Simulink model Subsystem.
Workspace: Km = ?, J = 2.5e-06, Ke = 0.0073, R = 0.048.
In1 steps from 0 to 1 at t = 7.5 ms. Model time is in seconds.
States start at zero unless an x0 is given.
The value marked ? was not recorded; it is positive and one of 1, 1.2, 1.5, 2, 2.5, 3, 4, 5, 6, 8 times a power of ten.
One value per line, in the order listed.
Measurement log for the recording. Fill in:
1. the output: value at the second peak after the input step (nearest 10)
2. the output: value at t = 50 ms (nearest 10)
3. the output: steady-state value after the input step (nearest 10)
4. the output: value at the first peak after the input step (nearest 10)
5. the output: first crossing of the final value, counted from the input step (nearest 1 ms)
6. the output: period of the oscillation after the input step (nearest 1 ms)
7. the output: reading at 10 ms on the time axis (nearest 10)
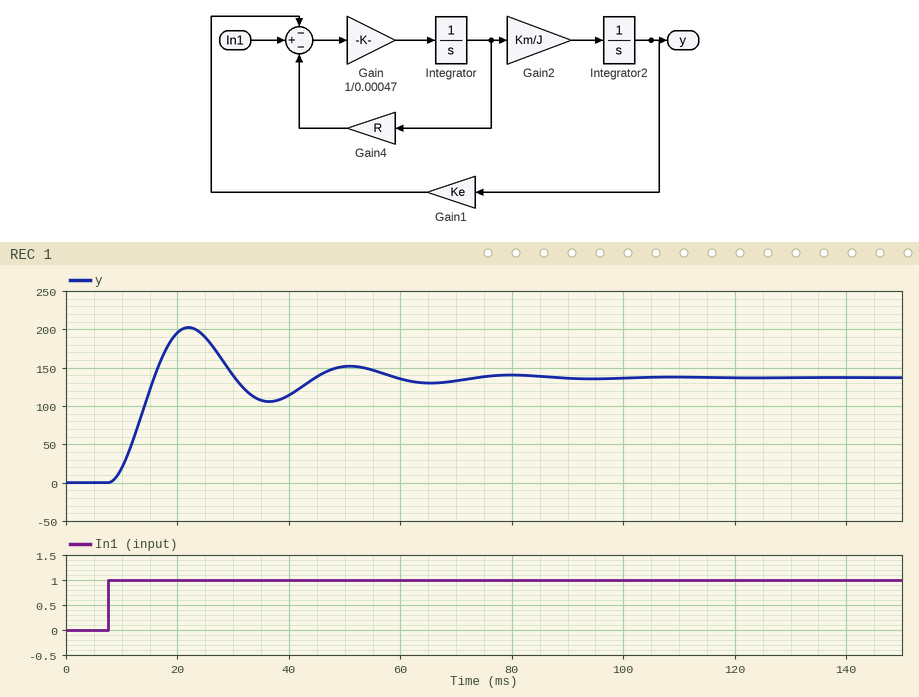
150
150
140
200
8 ms
29 ms
20
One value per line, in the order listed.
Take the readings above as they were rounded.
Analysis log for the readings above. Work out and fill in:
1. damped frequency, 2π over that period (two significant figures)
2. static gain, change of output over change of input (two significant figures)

0.22 rad/ms
140
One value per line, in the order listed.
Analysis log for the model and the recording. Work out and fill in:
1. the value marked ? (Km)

0.008
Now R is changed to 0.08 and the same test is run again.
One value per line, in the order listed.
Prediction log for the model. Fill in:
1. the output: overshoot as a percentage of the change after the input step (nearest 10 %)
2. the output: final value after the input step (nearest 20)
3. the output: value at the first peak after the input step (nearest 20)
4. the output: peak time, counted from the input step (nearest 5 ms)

30 %
140
180
15 ms
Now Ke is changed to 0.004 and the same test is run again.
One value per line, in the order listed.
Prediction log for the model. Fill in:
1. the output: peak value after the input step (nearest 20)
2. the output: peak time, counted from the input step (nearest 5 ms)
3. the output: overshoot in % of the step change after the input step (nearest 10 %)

340
20 ms
40 %
